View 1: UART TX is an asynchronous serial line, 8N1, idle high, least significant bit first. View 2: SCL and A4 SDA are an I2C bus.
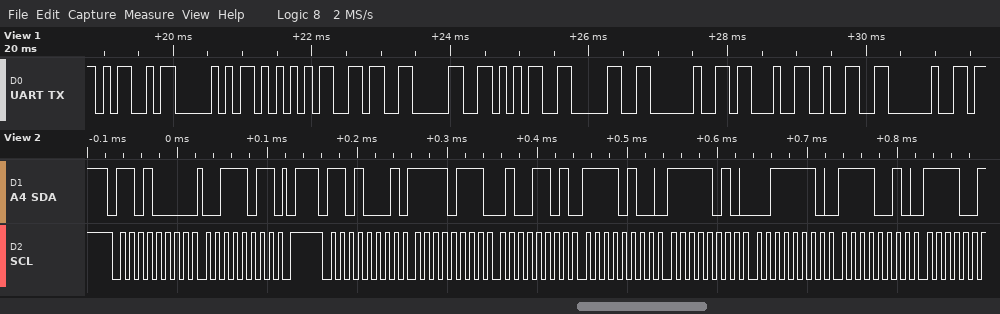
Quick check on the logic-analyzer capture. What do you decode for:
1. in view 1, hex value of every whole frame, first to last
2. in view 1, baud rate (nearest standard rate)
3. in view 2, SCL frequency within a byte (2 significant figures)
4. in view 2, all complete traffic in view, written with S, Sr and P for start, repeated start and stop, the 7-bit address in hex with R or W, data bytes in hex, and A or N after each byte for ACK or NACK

4D 50 55 36 30 35 30 20 23 32 20
9600 baud
100 kHz
S 68W A 3B A P S 68R A F7 A 4D A F4 A FA A 3E A F2 A
